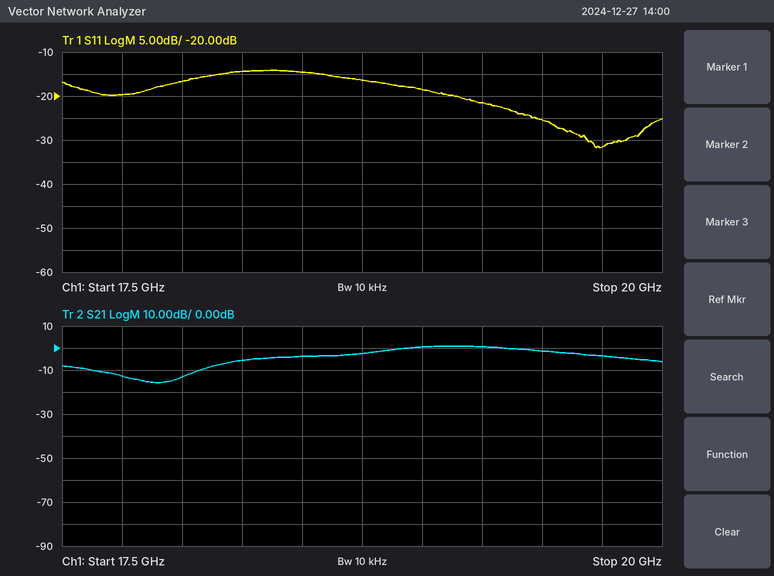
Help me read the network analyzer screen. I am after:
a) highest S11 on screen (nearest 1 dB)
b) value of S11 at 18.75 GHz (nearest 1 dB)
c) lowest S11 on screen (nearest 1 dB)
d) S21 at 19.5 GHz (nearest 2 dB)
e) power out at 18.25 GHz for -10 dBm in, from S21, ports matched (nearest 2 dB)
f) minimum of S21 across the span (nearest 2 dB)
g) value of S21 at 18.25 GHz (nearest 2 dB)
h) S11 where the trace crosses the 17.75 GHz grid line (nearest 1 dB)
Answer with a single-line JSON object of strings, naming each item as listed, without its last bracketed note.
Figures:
{"highest S11 on screen": "-14 dB", "value of S11 at 18.75 GHz": "-16 dB", "lowest S11 on screen": "-32 dB", "S21 at 19.5 GHz": "-2 dB", "power out at 18.25 GHz for -10 dBm in, from S21, ports matched": "-16 dBm", "minimum of S21 across the span": "-16 dB", "value of S21 at 18.25 GHz": "-6 dB", "S11 where the trace crosses the 17.75 GHz grid line": "-20 dB"}
